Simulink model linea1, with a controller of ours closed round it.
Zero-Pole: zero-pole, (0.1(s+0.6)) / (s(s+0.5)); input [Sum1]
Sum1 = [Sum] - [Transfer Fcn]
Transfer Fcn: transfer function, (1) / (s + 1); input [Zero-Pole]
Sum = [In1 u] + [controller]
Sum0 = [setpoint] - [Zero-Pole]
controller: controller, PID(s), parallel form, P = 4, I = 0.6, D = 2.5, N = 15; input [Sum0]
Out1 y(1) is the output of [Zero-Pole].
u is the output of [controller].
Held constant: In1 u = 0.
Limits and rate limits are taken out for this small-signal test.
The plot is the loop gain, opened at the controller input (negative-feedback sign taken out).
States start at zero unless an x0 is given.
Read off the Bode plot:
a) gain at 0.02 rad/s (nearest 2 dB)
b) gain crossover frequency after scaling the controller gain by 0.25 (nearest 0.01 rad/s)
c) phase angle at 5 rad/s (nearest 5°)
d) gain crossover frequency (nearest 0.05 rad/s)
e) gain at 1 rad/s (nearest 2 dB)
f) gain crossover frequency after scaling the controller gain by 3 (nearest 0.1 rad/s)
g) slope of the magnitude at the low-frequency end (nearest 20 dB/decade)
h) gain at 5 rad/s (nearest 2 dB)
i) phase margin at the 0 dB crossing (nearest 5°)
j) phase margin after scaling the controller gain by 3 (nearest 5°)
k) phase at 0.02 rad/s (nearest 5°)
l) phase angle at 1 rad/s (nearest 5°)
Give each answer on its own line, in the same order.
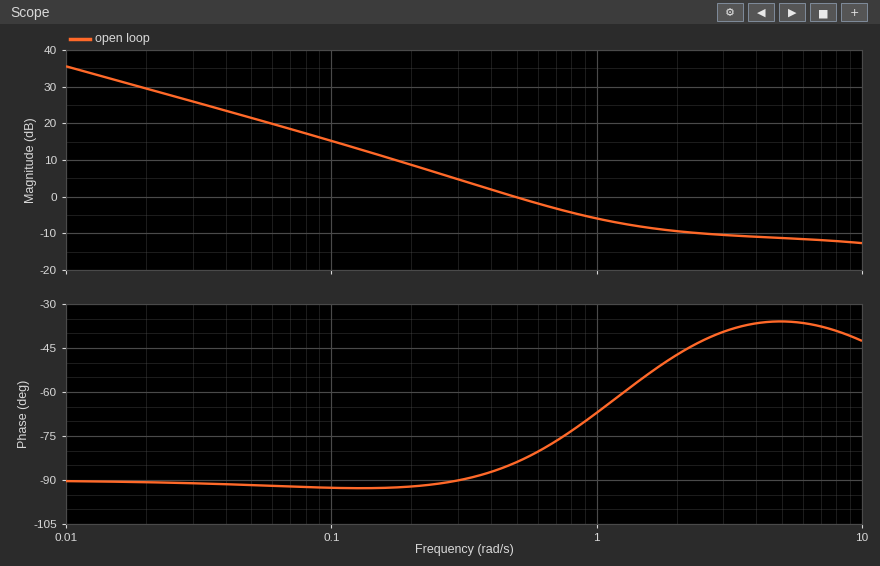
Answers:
30 dB
0.14 rad/s
-35°
0.50 rad/s
-6 dB
2.1 rad/s
-20 dB/decade
-12 dB
95°
135°
-90°
-65°
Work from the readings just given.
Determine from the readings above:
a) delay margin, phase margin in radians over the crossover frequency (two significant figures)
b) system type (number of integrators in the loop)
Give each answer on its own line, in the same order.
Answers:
3.3 s
1
